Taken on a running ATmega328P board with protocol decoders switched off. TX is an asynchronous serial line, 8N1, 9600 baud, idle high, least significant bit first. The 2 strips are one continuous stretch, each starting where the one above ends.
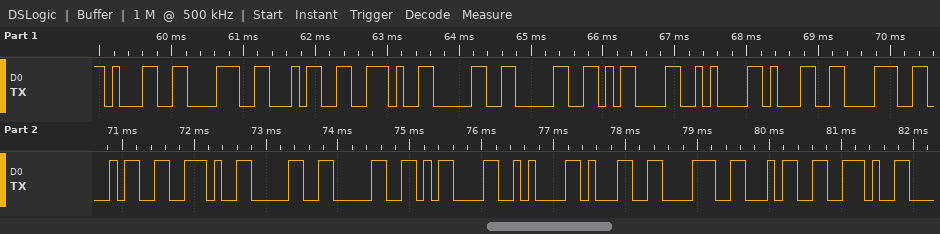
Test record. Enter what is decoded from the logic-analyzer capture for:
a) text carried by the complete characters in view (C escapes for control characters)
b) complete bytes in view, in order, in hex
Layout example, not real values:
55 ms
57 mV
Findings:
"184.00\r\n184.00\r\n184."
31 38 34 2E 30 30 0D 0A 31 38 34 2E 30 30 0D 0A 31 38 34 2E
